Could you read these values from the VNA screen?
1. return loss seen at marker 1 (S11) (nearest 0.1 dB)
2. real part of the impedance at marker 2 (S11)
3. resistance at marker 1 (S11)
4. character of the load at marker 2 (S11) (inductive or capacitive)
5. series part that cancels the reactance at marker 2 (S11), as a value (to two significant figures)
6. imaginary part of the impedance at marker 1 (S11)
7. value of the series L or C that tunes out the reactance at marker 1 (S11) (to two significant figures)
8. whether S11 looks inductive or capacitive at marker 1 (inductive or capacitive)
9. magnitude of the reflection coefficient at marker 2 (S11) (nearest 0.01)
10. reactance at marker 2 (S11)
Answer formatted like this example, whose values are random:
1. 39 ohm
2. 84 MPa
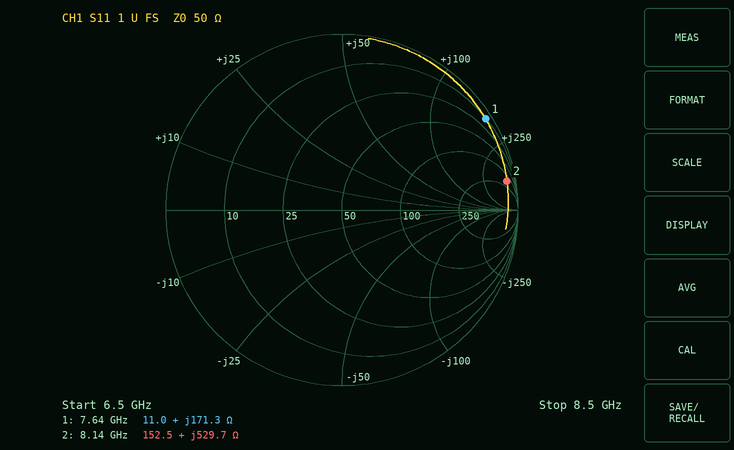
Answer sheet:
1. 0.3 dB
2. 152.5 Ω
3. 11.0 Ω
4. inductive
5. 37 fF
6. +171.3 Ω
7. 120 fF
8. inductive
9. 0.95
10. +529.7 Ω
